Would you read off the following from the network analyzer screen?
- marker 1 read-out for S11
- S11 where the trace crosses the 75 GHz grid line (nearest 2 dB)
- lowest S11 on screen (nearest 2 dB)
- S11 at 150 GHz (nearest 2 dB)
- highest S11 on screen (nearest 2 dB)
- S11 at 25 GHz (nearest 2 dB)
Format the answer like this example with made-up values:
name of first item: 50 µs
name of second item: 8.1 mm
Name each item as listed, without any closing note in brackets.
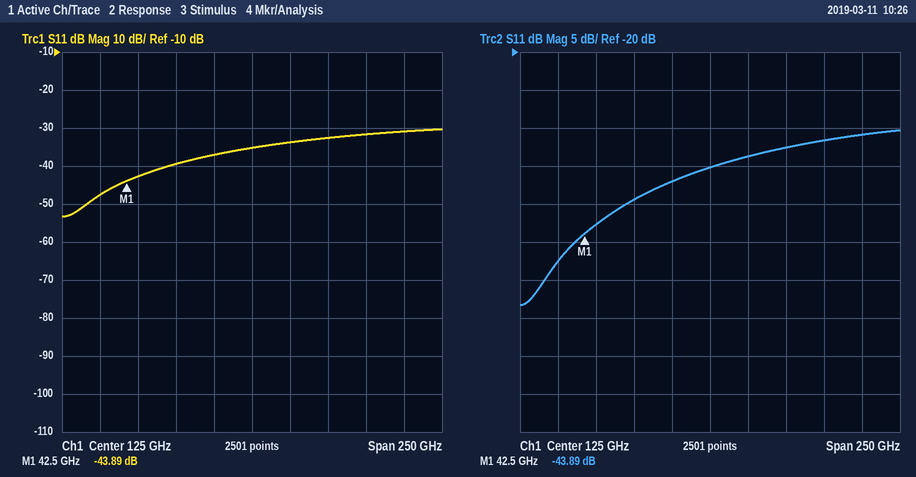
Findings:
marker 1 read-out for S11: -43.89 dB
S11 where the trace crosses the 75 GHz grid line: -40 dB
lowest S11 on screen: -54 dB
S11 at 150 GHz: -34 dB
highest S11 on screen: -30 dB
S11 at 25 GHz: -48 dB
